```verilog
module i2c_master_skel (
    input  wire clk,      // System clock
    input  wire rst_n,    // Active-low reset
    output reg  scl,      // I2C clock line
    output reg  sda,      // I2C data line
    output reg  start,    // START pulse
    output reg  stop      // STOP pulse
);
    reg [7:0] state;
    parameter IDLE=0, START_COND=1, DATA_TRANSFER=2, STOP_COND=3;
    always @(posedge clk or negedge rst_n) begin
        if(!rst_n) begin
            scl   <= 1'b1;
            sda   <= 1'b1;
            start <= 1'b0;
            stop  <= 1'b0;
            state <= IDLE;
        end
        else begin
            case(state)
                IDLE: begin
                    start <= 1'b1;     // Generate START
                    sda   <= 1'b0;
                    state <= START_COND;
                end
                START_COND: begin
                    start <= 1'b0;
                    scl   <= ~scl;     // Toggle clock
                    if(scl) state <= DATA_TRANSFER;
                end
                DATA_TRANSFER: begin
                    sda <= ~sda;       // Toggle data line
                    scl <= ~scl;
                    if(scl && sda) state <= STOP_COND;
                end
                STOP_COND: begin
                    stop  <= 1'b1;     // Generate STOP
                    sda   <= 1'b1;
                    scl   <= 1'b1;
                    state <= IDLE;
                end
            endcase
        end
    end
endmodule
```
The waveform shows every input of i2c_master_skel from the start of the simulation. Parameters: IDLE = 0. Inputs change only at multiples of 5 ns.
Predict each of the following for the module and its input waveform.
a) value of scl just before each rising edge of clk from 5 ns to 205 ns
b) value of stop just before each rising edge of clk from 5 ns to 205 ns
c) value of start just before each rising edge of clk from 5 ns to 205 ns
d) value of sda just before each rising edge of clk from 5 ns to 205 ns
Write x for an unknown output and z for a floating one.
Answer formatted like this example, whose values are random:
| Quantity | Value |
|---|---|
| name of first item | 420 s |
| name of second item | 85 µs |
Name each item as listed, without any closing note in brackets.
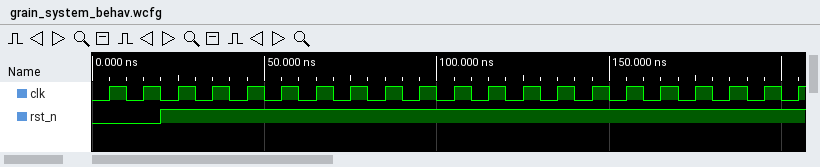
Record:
| Quantity | Value |
|---|---|
| value of scl just before each rising edge of clk from 5 ns to 205 ns | 1 1 1 1 0 1 0 1 1 0 1 0 1 1 0 1 0 1 1 0 1 |
| value of stop just before each rising edge of clk from 5 ns to 205 ns | 0 0 0 0 0 0 0 1 1 1 1 1 1 1 1 1 1 1 1 1 1 |
| value of start just before each rising edge of clk from 5 ns to 205 ns | 0 0 0 1 0 0 0 0 1 0 0 0 0 1 0 0 0 0 1 0 0 |
| value of sda just before each rising edge of clk from 5 ns to 205 ns | 1 1 1 0 0 1 0 1 0 0 1 0 1 0 0 1 0 1 0 0 1 |
